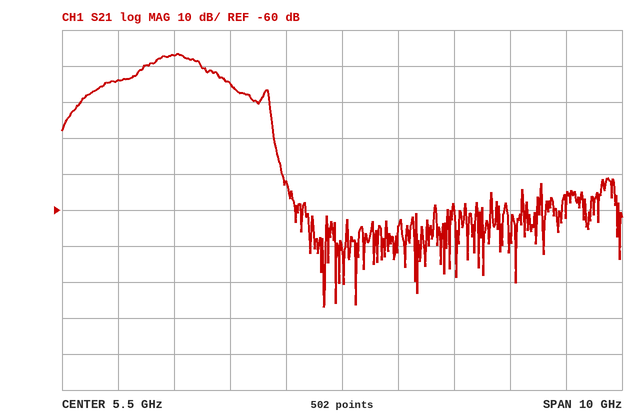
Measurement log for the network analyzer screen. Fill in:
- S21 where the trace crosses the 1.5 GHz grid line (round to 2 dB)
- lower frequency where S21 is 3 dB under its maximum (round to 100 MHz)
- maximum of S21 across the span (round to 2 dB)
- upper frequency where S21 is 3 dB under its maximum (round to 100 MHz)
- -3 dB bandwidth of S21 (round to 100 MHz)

-24 dB
2.1 GHz
-16 dB
3.0 GHz
900 MHz
